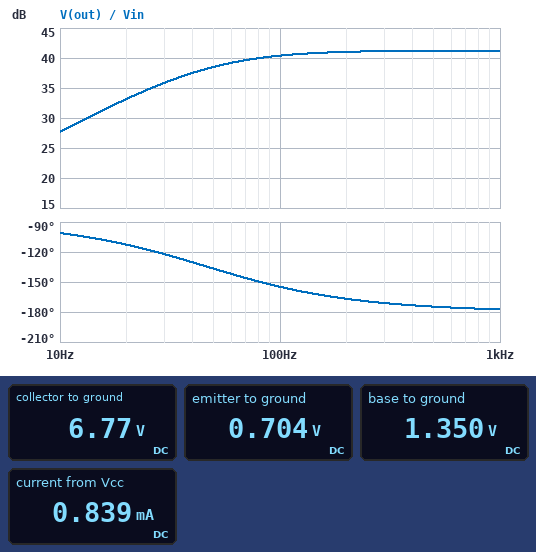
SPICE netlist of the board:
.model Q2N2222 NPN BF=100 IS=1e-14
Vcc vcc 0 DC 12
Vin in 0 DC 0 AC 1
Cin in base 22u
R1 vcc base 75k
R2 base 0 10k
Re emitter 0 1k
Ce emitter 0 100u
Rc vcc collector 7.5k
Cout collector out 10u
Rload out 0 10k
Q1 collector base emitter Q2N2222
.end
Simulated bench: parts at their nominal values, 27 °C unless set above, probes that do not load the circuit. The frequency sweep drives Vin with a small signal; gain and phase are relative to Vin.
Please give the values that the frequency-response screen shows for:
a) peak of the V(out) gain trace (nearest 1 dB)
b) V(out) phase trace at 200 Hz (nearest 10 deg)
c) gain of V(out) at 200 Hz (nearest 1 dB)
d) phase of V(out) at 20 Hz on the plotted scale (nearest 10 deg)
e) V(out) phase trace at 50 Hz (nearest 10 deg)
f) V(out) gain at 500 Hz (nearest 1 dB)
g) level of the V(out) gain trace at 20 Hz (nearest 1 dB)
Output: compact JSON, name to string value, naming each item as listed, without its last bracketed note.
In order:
{"peak of the V(out) gain trace": "41 dB", "V(out) phase trace at 200 Hz": "-170 deg", "gain of V(out) at 200 Hz": "41 dB", "phase of V(out) at 20 Hz on the plotted scale": "-110 deg", "V(out) phase trace at 50 Hz": "-140 deg", "V(out) gain at 500 Hz": "41 dB", "level of the V(out) gain trace at 20 Hz": "33 dB"}
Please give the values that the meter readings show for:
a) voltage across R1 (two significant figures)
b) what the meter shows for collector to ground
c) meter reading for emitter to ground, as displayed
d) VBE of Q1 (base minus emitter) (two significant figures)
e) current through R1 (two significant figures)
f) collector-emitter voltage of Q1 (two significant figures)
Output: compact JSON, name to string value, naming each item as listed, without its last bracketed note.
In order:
{"voltage across R1": "11 V", "what the meter shows for collector to ground": "6.77 V", "meter reading for emitter to ground, as displayed": "0.704 V", "VBE of Q1 (base minus emitter)": "650 mV", "current through R1": "140 µA", "collector-emitter voltage of Q1": "6.1 V"}
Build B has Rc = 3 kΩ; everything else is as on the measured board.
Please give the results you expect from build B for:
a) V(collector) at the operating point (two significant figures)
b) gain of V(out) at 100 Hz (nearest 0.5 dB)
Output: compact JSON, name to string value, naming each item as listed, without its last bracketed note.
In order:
{"V(collector) at the operating point": "9.9 V", "gain of V(out) at 100 Hz": "35.0 dB"}
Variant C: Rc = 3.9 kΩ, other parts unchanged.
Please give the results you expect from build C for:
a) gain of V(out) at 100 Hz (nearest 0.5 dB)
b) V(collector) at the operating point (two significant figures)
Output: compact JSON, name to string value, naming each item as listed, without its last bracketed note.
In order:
{"gain of V(out) at 100 Hz": "36.5 dB", "V(collector) at the operating point": "9.3 V"}
